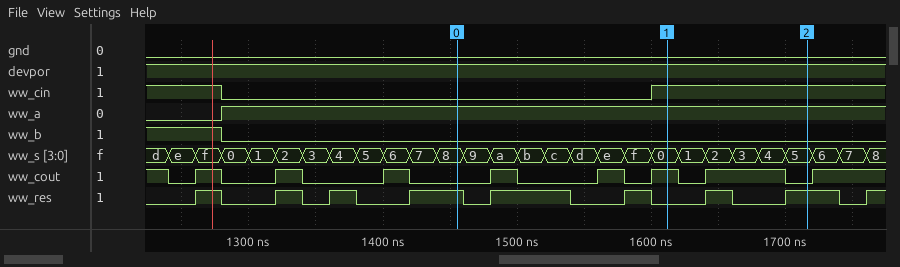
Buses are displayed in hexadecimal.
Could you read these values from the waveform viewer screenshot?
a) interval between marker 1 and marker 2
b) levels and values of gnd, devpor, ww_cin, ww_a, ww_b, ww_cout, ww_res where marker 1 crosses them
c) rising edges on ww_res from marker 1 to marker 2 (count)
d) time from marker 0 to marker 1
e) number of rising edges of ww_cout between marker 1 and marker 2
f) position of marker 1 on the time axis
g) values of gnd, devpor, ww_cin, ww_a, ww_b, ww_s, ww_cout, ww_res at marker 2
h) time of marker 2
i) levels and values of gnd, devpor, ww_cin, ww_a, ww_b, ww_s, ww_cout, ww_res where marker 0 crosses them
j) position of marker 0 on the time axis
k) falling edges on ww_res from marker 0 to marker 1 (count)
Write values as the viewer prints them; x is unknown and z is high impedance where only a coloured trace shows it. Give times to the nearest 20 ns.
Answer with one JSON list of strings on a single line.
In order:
["100 ns", "gnd=0, devpor=1, ww_cin=1, ww_a=1, ww_b=0, ww_cout=1, ww_res=0", "2", "160 ns", "1", "1620 ns", "gnd=0, devpor=1, ww_cin=1, ww_a=1, ww_b=0, ww_s=5, ww_cout=0, ww_res=1", "1720 ns", "gnd=0, devpor=1, ww_cin=0, ww_a=1, ww_b=0, ww_s=8, ww_cout=0, ww_res=1", "1460 ns", "3"]
